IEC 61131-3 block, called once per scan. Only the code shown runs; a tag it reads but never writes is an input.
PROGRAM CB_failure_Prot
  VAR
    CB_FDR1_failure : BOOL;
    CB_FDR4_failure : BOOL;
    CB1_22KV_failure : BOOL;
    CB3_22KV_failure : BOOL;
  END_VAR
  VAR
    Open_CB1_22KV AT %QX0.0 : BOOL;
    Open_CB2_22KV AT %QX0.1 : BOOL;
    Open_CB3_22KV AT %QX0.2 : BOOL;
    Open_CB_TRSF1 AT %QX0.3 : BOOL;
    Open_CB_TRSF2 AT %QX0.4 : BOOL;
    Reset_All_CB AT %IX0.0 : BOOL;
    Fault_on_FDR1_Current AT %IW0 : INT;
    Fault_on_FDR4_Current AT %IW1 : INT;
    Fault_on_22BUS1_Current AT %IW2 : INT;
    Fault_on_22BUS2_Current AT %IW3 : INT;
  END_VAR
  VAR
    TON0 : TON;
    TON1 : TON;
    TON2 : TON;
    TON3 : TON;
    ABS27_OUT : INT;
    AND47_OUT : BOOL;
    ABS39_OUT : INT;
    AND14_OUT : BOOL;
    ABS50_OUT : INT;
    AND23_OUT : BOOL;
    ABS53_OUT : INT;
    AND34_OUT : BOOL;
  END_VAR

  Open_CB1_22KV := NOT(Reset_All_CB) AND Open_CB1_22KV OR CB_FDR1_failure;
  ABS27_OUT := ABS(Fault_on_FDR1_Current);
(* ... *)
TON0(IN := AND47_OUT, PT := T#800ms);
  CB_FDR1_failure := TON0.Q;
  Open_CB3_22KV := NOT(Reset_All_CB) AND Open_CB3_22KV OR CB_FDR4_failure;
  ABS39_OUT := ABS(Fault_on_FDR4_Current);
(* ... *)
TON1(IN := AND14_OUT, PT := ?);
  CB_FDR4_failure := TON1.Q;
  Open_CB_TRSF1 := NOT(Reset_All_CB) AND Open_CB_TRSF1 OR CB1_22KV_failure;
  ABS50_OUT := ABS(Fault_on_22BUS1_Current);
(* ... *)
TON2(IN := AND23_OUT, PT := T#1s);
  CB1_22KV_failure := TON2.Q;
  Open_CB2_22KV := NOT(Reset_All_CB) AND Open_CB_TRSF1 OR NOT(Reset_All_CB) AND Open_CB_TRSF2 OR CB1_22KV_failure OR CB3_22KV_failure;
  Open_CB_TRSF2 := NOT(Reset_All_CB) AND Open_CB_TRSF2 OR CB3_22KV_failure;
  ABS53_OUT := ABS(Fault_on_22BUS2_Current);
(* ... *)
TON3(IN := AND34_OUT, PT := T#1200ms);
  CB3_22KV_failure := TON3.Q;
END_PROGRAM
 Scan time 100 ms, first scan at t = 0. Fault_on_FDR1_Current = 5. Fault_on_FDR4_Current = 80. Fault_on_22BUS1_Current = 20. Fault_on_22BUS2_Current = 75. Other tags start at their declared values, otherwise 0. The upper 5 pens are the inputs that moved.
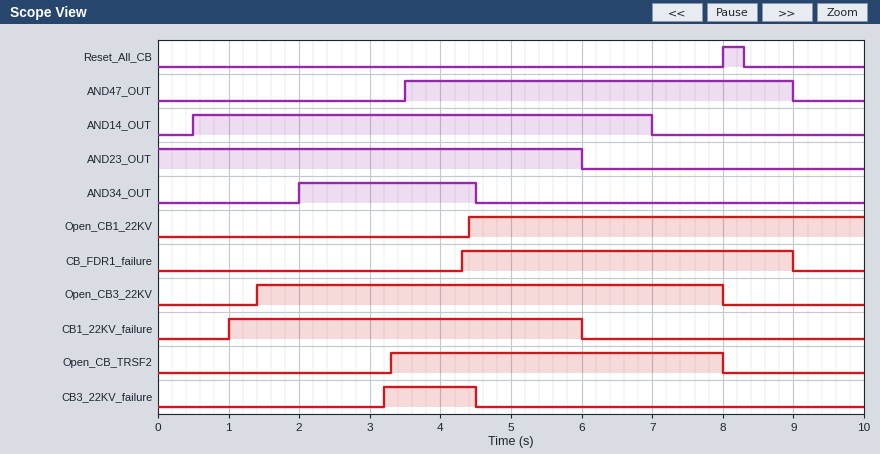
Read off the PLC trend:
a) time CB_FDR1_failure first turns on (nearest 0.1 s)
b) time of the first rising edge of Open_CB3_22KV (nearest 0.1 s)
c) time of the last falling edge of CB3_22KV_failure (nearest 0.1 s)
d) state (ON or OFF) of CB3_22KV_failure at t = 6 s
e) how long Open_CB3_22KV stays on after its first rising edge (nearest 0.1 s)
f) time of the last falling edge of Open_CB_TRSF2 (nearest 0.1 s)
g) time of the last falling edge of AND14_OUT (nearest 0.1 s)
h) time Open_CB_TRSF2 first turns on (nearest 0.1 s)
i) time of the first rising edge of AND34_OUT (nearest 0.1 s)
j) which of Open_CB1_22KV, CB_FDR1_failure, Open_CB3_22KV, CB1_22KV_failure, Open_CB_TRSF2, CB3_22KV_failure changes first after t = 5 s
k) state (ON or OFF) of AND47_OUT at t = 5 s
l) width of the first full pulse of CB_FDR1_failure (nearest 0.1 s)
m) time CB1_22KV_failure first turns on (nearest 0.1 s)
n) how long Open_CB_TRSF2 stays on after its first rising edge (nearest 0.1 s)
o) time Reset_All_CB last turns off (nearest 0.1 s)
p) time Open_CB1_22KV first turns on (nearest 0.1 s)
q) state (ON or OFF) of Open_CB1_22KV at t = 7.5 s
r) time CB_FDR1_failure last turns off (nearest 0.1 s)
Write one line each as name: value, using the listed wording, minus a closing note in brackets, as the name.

time CB_FDR1_failure first turns on: 4.3 s
time of the first rising edge of Open_CB3_22KV: 1.4 s
time of the last falling edge of CB3_22KV_failure: 4.5 s
state (ON or OFF) of CB3_22KV_failure at t = 6 s: OFF
how long Open_CB3_22KV stays on after its first rising edge: 6.6 s
time of the last falling edge of Open_CB_TRSF2: 8.0 s
time of the last falling edge of AND14_OUT: 7.0 s
time Open_CB_TRSF2 first turns on: 3.3 s
time of the first rising edge of AND34_OUT: 2.0 s
which of Open_CB1_22KV, CB_FDR1_failure, Open_CB3_22KV, CB1_22KV_failure, Open_CB_TRSF2, CB3_22KV_failure changes first after t = 5 s: CB1_22KV_failure
state (ON or OFF) of AND47_OUT at t = 5 s: ON
width of the first full pulse of CB_FDR1_failure: 4.7 s
time CB1_22KV_failure first turns on: 1.0 s
how long Open_CB_TRSF2 stays on after its first rising edge: 4.7 s
time Reset_All_CB last turns off: 8.3 s
time Open_CB1_22KV first turns on: 4.4 s
state (ON or OFF) of Open_CB1_22KV at t = 7.5 s: ON
time CB_FDR1_failure last turns off: 9.0 s
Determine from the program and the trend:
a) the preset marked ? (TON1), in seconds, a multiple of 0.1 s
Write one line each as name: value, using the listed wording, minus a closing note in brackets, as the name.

the preset marked ? (TON1), in seconds, a multiple of 0.1 s: 0.8 s
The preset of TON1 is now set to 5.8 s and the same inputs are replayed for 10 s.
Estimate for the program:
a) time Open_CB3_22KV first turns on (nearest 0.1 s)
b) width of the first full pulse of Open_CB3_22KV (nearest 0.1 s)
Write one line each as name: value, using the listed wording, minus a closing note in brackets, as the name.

time Open_CB3_22KV first turns on: 6.4 s
width of the first full pulse of Open_CB3_22KV: 1.6 s
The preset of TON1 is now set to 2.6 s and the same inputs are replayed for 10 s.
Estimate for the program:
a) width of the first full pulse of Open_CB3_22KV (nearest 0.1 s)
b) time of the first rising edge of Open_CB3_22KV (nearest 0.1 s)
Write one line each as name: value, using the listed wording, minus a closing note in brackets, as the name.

width of the first full pulse of Open_CB3_22KV: 4.8 s
time of the first rising edge of Open_CB3_22KV: 3.2 s
